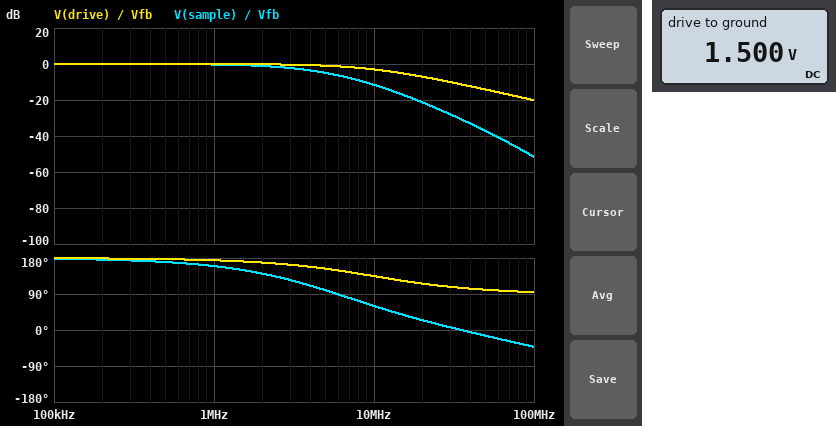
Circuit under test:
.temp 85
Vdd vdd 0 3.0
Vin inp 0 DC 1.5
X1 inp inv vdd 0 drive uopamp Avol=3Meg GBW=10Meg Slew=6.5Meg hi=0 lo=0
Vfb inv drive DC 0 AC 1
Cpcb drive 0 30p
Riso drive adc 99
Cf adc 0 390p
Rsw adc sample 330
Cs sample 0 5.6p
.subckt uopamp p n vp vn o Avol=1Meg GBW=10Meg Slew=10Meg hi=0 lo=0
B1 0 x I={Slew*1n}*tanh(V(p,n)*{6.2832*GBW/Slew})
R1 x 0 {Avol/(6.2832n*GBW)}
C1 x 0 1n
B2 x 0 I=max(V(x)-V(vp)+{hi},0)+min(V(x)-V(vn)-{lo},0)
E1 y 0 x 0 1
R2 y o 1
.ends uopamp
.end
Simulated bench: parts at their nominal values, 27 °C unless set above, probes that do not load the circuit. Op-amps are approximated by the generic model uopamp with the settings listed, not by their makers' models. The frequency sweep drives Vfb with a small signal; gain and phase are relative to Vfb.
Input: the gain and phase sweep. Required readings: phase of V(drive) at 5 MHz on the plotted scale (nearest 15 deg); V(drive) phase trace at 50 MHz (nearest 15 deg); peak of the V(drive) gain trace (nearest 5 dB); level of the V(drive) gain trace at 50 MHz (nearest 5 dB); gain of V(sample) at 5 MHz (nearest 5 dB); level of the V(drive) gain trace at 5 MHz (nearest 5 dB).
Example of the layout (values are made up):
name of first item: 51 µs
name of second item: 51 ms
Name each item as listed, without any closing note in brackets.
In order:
phase of V(drive) at 5 MHz on the plotted scale: 150 deg
V(drive) phase trace at 50 MHz: 105 deg
peak of the V(drive) gain trace: 0 dB
level of the V(drive) gain trace at 50 MHz: -15 dB
gain of V(sample) at 5 MHz: -5 dB
level of the V(drive) gain trace at 5 MHz: 0 dB
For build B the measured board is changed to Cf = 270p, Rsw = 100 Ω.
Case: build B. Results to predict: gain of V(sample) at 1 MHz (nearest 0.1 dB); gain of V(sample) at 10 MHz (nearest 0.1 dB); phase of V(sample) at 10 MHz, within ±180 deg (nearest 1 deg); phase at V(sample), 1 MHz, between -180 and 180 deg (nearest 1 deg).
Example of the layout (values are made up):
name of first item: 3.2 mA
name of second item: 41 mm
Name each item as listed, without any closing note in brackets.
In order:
gain of V(sample) at 1 MHz: -0.2 dB
gain of V(sample) at 10 MHz: -9.0 dB
phase of V(sample) at 10 MHz, within ±180 deg: 73 deg
phase at V(sample), 1 MHz, between -180 and 180 deg: 164 deg
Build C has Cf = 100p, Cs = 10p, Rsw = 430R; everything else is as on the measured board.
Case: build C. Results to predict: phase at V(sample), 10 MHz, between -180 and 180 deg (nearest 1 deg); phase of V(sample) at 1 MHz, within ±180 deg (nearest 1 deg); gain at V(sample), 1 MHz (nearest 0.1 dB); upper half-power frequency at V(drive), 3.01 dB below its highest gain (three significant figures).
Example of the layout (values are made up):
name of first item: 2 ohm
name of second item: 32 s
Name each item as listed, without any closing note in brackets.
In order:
phase at V(sample), 10 MHz, between -180 and 180 deg: 86 deg
phase of V(sample) at 1 MHz, within ±180 deg: 169 deg
gain at V(sample), 1 MHz: -0.1 dB
upper half-power frequency at V(drive), 3.01 dB below its highest gain: 10.0 MHz
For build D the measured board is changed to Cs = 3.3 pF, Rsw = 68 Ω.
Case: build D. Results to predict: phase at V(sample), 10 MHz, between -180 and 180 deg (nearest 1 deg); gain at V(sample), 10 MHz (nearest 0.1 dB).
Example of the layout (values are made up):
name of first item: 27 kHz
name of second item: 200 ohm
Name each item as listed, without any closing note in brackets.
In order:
phase at V(sample), 10 MHz, between -180 and 180 deg: 66 deg
gain at V(sample), 10 MHz: -11.5 dB
